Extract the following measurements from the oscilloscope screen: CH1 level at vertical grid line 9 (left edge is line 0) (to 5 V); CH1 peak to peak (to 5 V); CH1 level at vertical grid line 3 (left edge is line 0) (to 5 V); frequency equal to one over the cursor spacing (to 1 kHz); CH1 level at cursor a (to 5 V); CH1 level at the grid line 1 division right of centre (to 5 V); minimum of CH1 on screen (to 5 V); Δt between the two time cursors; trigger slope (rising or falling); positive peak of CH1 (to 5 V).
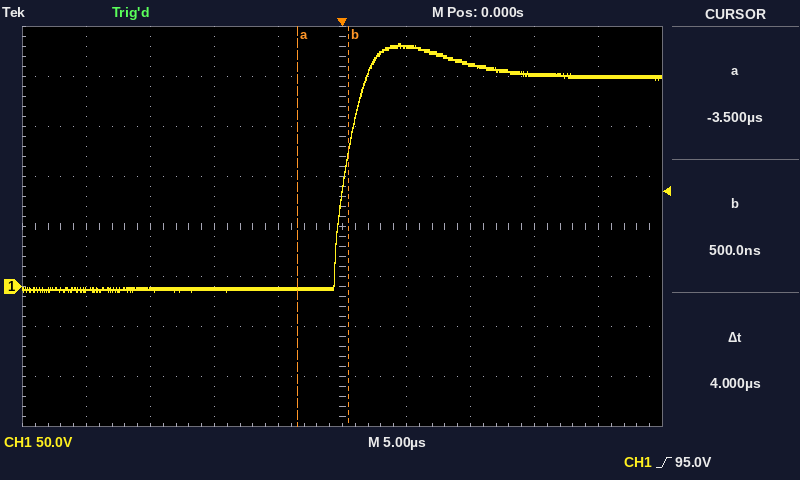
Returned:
210 V
250 V
0 V
250 kHz
0 V
240 V
-5 V
4 µs
rising
245 V
